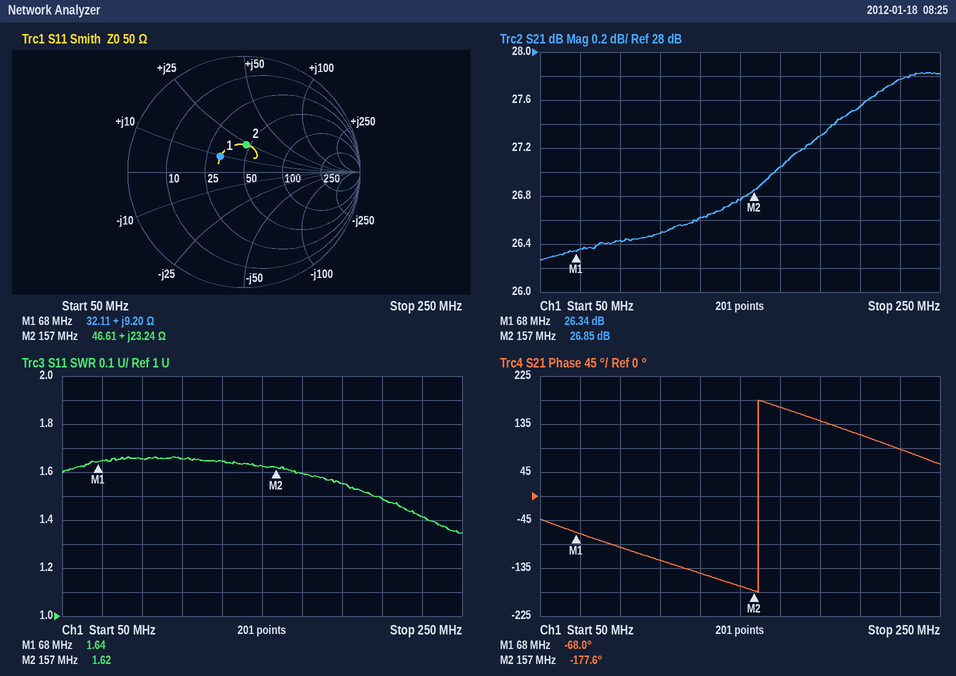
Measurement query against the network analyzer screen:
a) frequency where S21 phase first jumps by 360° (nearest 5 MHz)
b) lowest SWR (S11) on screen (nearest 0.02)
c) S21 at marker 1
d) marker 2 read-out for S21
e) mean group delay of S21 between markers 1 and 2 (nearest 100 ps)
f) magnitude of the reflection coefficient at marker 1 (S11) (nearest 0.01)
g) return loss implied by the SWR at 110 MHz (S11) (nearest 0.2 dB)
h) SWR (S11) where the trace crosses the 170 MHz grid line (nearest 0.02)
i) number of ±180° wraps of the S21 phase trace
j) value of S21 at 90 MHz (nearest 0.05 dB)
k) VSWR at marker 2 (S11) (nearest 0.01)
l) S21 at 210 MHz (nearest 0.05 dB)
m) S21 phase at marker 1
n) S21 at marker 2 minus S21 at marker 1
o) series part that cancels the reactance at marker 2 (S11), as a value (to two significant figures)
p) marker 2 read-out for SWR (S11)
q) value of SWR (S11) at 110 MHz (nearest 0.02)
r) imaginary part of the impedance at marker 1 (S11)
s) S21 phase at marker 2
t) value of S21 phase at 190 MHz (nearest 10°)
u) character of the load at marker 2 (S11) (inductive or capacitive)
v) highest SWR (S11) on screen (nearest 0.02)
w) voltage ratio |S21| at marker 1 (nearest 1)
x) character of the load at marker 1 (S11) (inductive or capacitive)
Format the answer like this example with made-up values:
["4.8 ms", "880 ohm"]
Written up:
["160 MHz", "1.34", "26.34 dB", "26.85 dB", "3.4 ns", "0.24", "12.2 dB", "1.60", "1", "26.45 dB", "1.62", "27.55 dB", "-68.0°", "0.51 dB", "44 pF", "1.62", "1.66", "+9.20 Ω", "-177.6°", "140°", "inductive", "1.66", "21", "inductive"]
